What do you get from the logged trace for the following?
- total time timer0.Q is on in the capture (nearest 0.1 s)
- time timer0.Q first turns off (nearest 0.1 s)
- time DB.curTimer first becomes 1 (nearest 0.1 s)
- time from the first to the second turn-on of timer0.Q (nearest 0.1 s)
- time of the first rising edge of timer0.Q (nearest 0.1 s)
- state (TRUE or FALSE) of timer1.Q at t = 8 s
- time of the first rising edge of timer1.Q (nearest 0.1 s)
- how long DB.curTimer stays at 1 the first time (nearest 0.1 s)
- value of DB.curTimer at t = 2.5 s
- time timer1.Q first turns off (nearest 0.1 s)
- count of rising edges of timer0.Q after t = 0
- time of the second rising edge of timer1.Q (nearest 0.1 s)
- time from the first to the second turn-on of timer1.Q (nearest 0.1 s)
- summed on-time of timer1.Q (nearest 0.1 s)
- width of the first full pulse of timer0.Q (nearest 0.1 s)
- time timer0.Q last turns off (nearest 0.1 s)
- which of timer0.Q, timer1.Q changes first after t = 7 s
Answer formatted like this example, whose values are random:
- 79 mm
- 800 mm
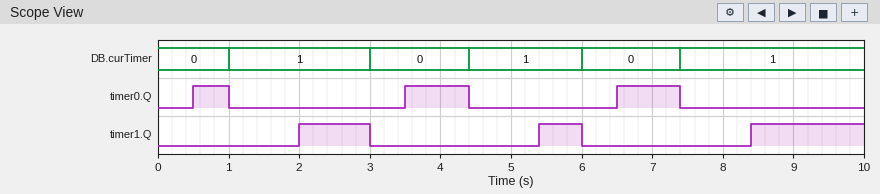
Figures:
- 2.3 s
- 1.0 s
- 1.0 s
- 3.0 s
- 0.5 s
- FALSE
- 2.0 s
- 2.0 s
- 1
- 3.0 s
- 3
- 5.4 s
- 3.4 s
- 3.2 s
- 0.5 s
- 7.4 s
- timer0.Q
